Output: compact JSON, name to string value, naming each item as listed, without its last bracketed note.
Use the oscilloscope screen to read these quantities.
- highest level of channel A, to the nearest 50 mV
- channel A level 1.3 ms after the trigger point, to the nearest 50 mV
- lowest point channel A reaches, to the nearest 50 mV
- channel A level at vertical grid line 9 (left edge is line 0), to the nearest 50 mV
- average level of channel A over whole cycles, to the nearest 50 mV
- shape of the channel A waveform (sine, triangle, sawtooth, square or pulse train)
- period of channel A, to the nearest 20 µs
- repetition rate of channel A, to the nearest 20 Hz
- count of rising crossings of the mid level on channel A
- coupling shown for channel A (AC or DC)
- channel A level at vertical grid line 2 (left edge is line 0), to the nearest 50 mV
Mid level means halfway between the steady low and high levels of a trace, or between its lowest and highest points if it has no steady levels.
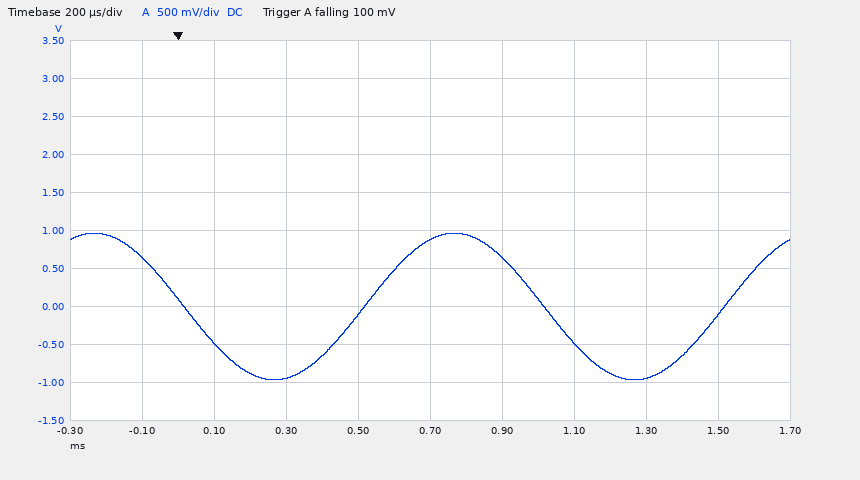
{"highest level of channel A, to the nearest 50 mV": "950 mV", "channel A level 1.3 ms after the trigger point, to the nearest 50 mV": "-950 mV", "lowest point channel A reaches, to the nearest 50 mV": "-950 mV", "channel A level at vertical grid line 9 (left edge is line 0), to the nearest 50 mV": "-100 mV", "average level of channel A over whole cycles, to the nearest 50 mV": "0 mV", "shape of the channel A waveform": "sine", "period of channel A, to the nearest 20 µs": "1.00 ms", "repetition rate of channel A, to the nearest 20 Hz": "1.00 kHz", "count of rising crossings of the mid level on channel A": "2", "coupling shown for channel A": "DC", "channel A level at vertical grid line 2 (left edge is line 0), to the nearest 50 mV": "-500 mV"}
